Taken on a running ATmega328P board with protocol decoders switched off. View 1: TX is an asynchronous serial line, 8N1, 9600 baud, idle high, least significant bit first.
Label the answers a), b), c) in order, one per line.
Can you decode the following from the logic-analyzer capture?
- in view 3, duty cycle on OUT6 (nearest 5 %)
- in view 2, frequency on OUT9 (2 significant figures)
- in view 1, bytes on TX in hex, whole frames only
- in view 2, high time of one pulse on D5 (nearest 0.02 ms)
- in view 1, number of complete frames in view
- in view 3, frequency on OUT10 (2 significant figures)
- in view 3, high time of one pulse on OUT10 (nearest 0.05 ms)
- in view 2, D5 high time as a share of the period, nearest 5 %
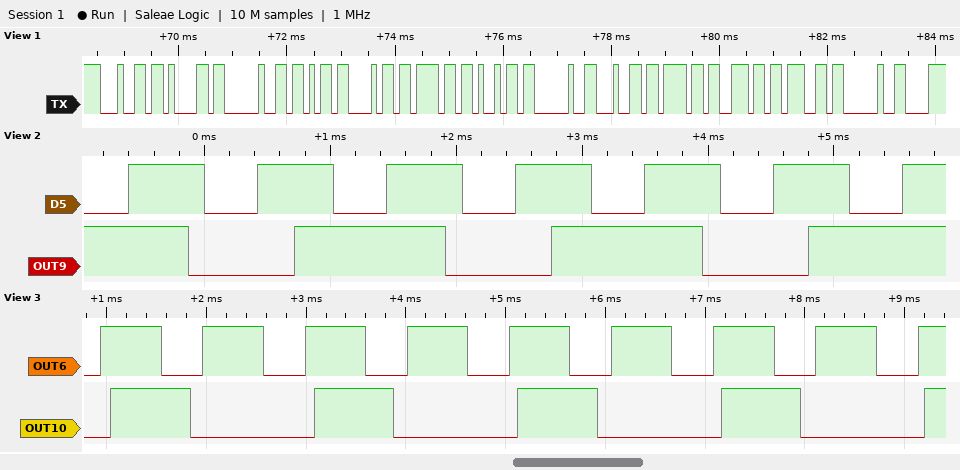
a) 60 %
b) 490 Hz
c) 0x64 0x61 0x20 0x6B 0x68 0x6F 0x69 0x20 0x64 0x6F 0x6E 0x67 0x20
d) 0.60 ms
e) 13
f) 490 Hz
g) 0.80 ms
h) 60 %
